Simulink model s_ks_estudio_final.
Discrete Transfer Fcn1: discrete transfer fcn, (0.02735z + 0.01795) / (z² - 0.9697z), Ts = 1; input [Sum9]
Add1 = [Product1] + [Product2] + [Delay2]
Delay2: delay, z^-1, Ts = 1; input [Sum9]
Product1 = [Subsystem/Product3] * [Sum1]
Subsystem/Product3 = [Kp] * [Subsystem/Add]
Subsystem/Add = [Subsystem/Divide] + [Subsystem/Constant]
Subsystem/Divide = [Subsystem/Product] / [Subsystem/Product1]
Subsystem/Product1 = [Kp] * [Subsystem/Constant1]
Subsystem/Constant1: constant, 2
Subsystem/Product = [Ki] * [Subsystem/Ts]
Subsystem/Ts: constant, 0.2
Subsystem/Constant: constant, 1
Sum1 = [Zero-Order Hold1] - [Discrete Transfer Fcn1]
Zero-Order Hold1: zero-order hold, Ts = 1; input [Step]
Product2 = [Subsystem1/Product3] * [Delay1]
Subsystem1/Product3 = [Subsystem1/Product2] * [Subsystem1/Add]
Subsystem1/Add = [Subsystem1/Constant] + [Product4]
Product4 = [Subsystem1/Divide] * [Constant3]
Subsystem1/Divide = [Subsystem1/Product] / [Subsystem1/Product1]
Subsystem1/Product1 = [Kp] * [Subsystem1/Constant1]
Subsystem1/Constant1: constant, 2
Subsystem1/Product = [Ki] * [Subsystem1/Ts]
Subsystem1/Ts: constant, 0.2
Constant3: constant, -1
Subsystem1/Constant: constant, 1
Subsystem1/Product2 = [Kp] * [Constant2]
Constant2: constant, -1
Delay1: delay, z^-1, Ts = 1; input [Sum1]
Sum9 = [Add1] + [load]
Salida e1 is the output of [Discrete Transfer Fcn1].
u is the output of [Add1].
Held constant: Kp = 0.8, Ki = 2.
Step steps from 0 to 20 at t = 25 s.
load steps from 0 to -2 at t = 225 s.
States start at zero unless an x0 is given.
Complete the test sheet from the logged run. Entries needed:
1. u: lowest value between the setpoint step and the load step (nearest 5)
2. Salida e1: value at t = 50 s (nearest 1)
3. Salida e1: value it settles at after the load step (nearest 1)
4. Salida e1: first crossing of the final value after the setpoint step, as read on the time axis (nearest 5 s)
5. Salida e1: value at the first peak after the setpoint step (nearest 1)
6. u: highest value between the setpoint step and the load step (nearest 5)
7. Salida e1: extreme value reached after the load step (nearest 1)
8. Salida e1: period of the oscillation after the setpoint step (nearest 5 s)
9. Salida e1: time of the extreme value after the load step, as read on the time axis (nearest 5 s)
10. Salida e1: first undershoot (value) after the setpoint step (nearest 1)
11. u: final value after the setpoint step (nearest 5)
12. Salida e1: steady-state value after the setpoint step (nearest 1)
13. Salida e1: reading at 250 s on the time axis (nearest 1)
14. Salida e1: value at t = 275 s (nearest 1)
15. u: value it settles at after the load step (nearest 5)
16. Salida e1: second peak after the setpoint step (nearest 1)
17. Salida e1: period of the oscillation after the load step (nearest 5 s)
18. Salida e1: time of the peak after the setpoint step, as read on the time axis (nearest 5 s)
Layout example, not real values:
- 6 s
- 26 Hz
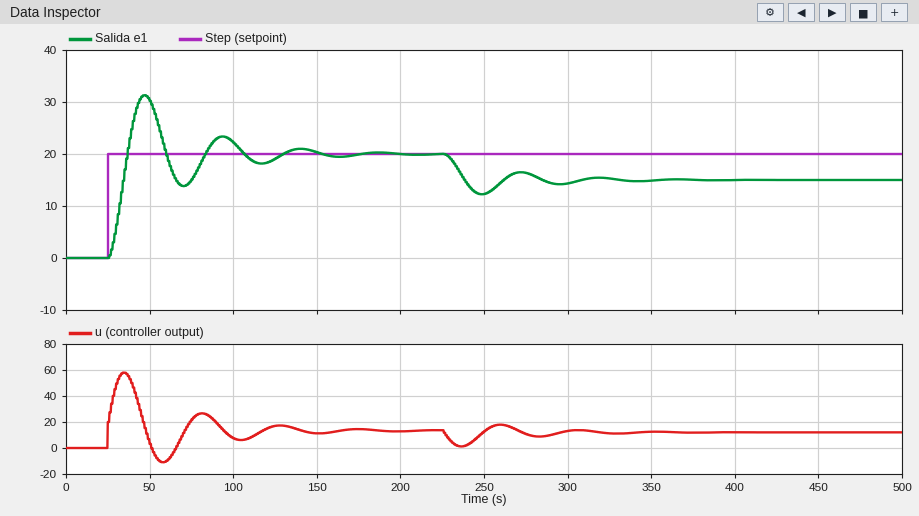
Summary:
- -10
- 30
- 15
- 35 s
- 31
- 60
- 12
- 45 s
- 250 s
- 14
- 15
- 20
- 12
- 16
- 10
- 23
- 45 s
- 45 s
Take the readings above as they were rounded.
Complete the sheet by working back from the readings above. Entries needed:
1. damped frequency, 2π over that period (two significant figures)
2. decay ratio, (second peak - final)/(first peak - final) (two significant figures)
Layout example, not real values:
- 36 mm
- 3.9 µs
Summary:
- 0.14 rad/s
- 0.27
